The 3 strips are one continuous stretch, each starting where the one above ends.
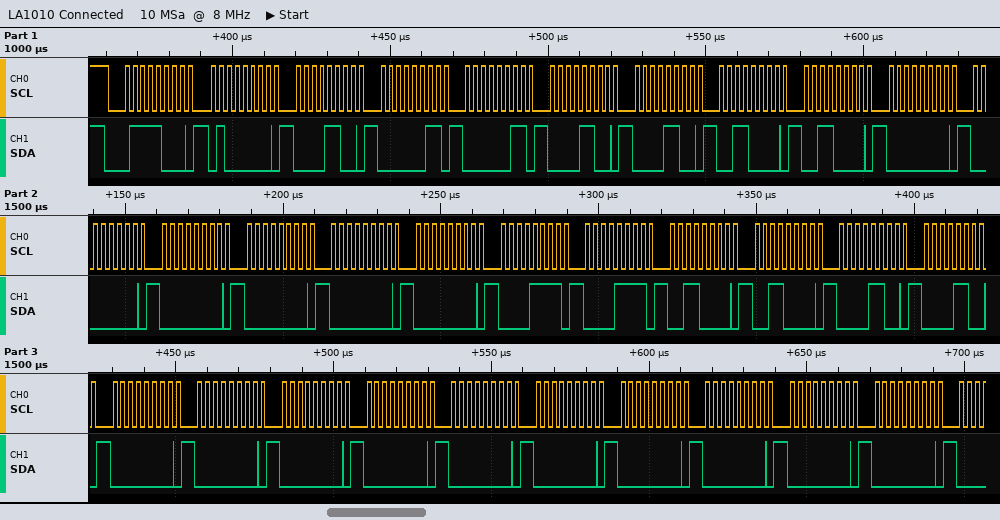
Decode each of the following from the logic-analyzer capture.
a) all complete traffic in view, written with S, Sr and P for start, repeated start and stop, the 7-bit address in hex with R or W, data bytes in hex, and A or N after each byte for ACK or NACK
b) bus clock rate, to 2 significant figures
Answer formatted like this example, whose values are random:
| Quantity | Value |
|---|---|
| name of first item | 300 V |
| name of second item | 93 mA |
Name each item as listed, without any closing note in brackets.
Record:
| Quantity | Value |
|---|---|
| all complete traffic in view, written with S, Sr and P for start, repeated start and stop, the 7-bit address in hex with R or W, data bytes in hex, and A or N after each byte for ACK or NACK | S 3CW A 40 A 0C A 03 A 03 A 0C A 0C A 30 A 30 A 00 A 00 A 00 A 00 A 00 A 00 A 0F A 0F A 30 A 30 A 0C A 0C A 00 A 00 A 00 A 00 A 00 A 00 A 00 A 00 A 00 A 00 A |
| bus clock rate, to 2 significant figures | 400 kHz |
